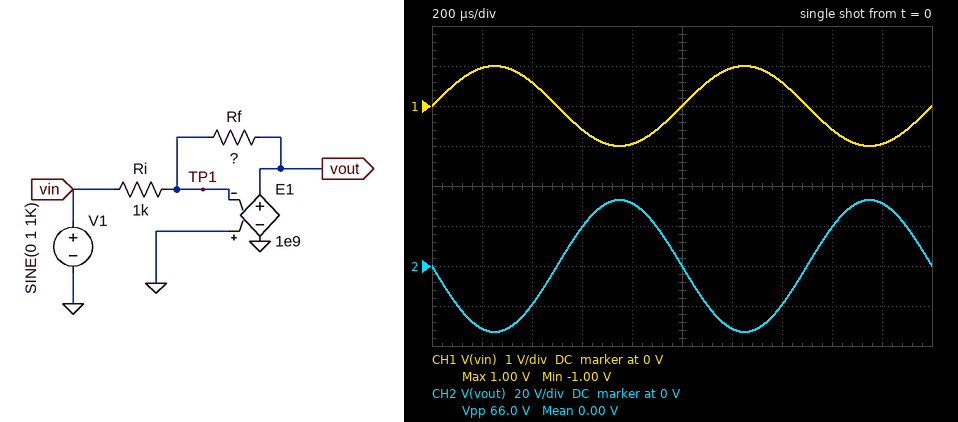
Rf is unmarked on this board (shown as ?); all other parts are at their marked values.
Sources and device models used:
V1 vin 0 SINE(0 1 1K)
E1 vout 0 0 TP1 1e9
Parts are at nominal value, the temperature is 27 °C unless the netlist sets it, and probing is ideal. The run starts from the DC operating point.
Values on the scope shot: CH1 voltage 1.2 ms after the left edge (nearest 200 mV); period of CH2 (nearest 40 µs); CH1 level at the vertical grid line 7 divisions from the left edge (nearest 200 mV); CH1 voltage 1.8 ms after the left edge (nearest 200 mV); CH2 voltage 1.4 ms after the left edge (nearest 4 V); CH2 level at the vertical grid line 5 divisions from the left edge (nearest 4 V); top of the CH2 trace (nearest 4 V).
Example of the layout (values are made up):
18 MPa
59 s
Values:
1.0 V
1.00 ms
600 mV
-1.0 V
-20 V
0 V
32 V
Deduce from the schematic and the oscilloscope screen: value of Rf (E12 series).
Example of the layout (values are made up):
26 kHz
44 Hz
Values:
33 kΩ
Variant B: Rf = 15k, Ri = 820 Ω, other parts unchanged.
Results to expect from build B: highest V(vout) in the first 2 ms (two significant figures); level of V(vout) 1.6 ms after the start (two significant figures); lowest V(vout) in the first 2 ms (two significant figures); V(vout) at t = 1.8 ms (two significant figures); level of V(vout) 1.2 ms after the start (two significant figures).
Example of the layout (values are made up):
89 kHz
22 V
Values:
18 V
11 V
-18 V
17 V
-17 V
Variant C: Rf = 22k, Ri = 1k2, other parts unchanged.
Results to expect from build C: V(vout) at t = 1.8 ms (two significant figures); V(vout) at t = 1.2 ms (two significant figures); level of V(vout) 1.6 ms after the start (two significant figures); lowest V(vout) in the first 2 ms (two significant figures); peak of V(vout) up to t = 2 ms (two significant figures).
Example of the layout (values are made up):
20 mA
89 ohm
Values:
17 V
-17 V
11 V
-18 V
18 V
